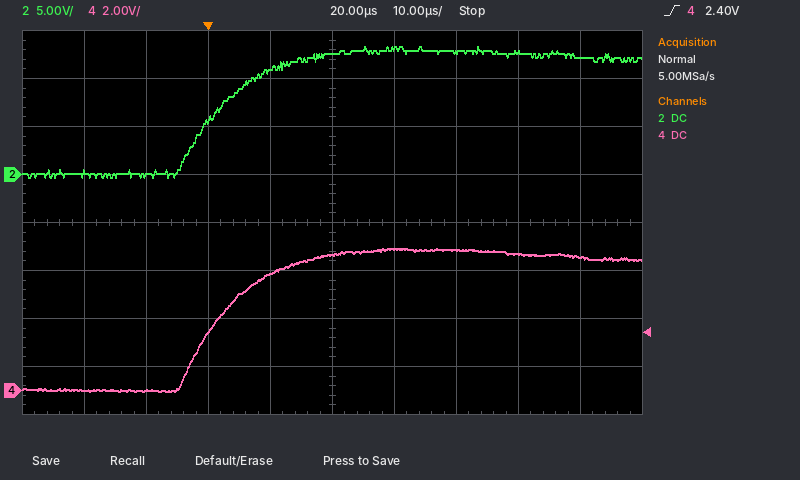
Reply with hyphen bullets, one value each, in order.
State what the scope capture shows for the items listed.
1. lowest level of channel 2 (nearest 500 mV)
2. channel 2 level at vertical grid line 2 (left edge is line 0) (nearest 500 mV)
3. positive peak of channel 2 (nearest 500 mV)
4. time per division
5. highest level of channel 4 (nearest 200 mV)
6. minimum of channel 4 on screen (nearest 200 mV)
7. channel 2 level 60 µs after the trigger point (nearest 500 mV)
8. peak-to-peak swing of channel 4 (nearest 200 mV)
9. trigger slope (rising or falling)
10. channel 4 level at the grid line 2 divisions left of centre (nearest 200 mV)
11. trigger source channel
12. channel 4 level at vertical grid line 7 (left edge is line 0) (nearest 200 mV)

- -500 mV
- 0.0 V
- 13.5 V
- 10 µs
- 6.0 V
- 0.0 V
- 12.0 V
- 6.0 V
- rising
- 2.4 V
- channel 4
- 5.8 V
